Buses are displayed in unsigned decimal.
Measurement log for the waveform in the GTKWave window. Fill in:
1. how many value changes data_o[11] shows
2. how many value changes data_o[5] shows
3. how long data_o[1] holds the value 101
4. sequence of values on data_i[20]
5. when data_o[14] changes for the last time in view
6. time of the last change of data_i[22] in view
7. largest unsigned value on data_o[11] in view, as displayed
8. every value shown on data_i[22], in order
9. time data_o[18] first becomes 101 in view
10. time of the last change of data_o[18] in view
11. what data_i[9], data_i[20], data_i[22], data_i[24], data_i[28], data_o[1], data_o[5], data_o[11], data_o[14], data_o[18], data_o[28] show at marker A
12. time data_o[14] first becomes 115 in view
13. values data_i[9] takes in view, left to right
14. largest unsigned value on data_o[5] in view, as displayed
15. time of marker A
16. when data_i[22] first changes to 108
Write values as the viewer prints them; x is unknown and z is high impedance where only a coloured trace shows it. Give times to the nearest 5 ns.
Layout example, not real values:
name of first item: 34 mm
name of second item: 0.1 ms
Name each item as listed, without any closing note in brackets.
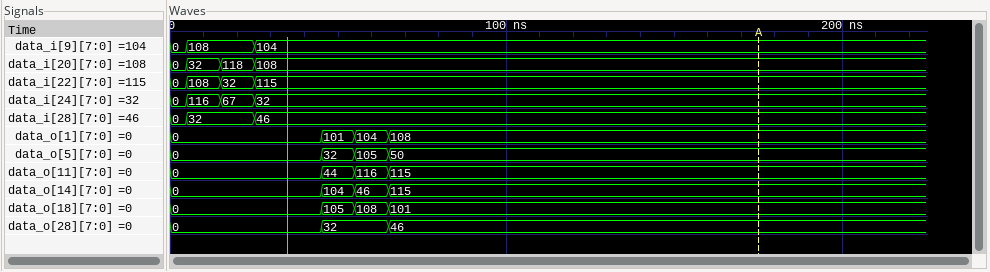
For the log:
how many value changes data_o[11] shows: 3
how many value changes data_o[5] shows: 3
how long data_o[1] holds the value 101: 10 ns
sequence of values on data_i[20]: 0, 32, 118, 108
when data_o[14] changes for the last time in view: 65 ns
time of the last change of data_i[22] in view: 25 ns
largest unsigned value on data_o[11] in view, as displayed: 116
every value shown on data_i[22], in order: 0, 108, 32, 115
time data_o[18] first becomes 101 in view: 65 ns
time of the last change of data_o[18] in view: 65 ns
what data_i[9], data_i[20], data_i[22], data_i[24], data_i[28], data_o[1], data_o[5], data_o[11], data_o[14], data_o[18], data_o[28] show at marker A: data_i[9]=104, data_i[20]=108, data_i[22]=115, data_i[24]=32, data_i[28]=46, data_o[1]=108, data_o[5]=50, data_o[11]=115, data_o[14]=115, data_o[18]=101, data_o[28]=46
time data_o[14] first becomes 115 in view: 65 ns
values data_i[9] takes in view, left to right: 0, 108, 104
largest unsigned value on data_o[5] in view, as displayed: 105
time of marker A: 175 ns
when data_i[22] first changes to 108: 5 ns
